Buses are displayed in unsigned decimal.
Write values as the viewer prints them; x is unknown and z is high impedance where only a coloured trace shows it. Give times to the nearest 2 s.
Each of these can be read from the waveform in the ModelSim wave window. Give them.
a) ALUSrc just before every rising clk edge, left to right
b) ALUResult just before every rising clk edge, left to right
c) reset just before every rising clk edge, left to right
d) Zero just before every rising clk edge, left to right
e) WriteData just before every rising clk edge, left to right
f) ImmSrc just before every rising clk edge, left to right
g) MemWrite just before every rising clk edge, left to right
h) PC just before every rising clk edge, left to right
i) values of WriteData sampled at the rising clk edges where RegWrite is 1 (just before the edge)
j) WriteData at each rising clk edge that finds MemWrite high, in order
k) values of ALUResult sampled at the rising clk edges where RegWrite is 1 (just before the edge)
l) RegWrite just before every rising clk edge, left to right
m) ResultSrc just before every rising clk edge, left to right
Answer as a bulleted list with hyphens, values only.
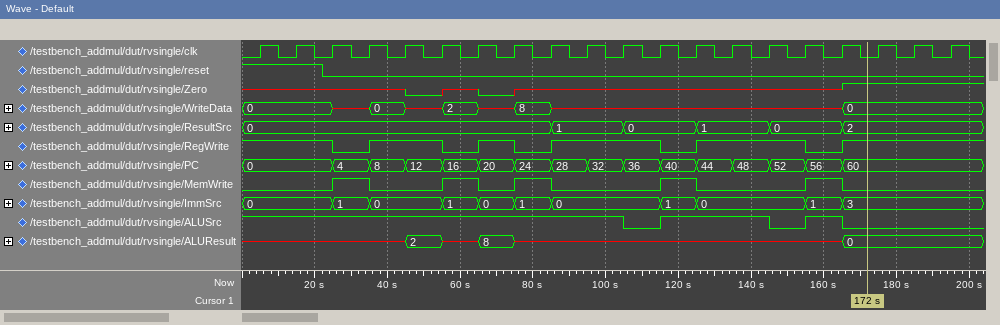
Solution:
- 1 1 1 1 1 1 1 1 1 1 1 0 1 1 1 0 1 0 0 0
- x, x, x, x, x, 2, x, 8, x, x, x, x, x, x, x, x, x, 0, 0, 0
- 1 1 0 0 0 0 0 0 0 0 0 0 0 0 0 0 0 0 0 0
- x x x x x 0 x 0 x x x x x x x x x 1 1 1
- 0, 0, 0, x, 0, x, 2, x, 8, x, x, x, x, x, x, x, x, 0, 0, 0
- 0, 0, 0, 1, 0, 0, 1, 0, 1, 0, 0, 0, 1, 0, 0, 0, 1, 3, 3, 3
- 0 0 0 1 0 0 1 0 1 0 0 0 1 0 0 0 1 0 0 0
- 0, 0, 0, 4, 8, 12, 16, 20, 24, 28, 32, 36, 40, 44, 48, 52, 56, 60, 60, 60
- 0, 0, 0, 0, x, x, x, x, x, x, x, x, 0, 0, 0
- x, 2, 8, x, x
- x, x, x, x, 2, 8, x, x, x, x, x, x, 0, 0, 0
- 1 1 1 0 1 1 0 1 0 1 1 1 0 1 1 1 0 1 1 1
- 0, 0, 0, 0, 0, 0, 0, 0, 0, 1, 1, 0, 0, 1, 1, 0, 0, 2, 2, 2
